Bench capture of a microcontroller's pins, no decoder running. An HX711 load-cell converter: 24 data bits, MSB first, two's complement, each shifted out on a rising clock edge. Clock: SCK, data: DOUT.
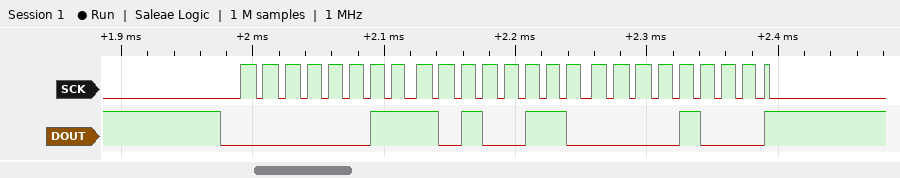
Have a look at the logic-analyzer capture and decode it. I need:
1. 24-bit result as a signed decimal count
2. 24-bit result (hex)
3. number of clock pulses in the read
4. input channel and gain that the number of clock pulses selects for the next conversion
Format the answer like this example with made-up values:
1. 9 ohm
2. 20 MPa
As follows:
1. 239112
2. 0x03A608
3. 25
4. channel A, gain 128
